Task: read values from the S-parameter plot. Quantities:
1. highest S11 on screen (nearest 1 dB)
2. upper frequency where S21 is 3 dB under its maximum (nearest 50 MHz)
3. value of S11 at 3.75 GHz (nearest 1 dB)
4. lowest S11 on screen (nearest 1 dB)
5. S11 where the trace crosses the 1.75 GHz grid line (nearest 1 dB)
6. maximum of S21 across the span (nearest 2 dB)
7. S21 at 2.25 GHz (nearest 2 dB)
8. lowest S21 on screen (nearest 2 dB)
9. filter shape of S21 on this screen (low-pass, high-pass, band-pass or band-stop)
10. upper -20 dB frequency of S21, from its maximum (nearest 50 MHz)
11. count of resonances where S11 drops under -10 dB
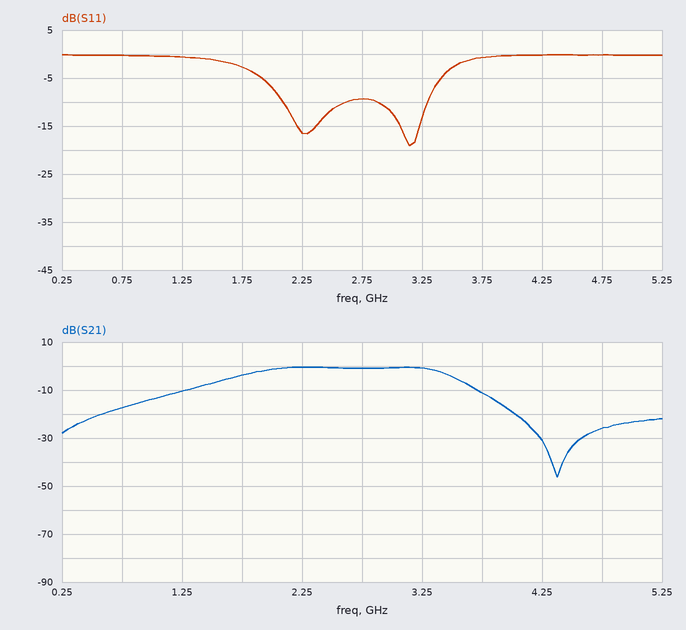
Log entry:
0 dB
3.45 GHz
-1 dB
-19 dB
-3 dB
0 dB
0 dB
-46 dB
band-pass
4.05 GHz
2
